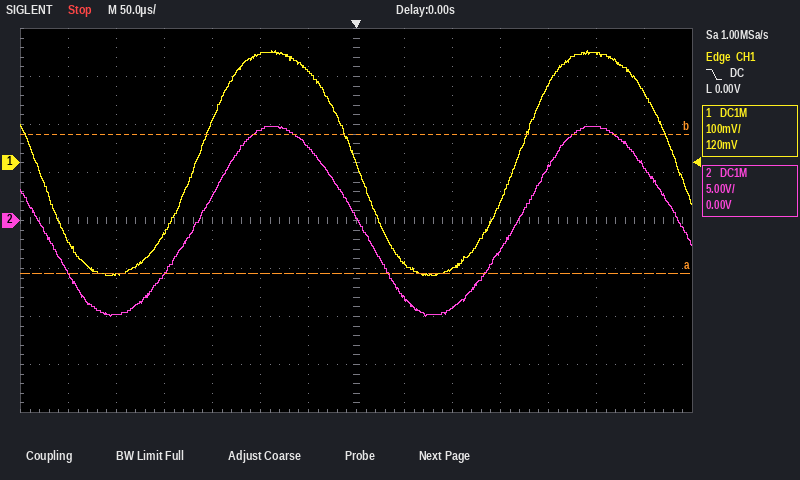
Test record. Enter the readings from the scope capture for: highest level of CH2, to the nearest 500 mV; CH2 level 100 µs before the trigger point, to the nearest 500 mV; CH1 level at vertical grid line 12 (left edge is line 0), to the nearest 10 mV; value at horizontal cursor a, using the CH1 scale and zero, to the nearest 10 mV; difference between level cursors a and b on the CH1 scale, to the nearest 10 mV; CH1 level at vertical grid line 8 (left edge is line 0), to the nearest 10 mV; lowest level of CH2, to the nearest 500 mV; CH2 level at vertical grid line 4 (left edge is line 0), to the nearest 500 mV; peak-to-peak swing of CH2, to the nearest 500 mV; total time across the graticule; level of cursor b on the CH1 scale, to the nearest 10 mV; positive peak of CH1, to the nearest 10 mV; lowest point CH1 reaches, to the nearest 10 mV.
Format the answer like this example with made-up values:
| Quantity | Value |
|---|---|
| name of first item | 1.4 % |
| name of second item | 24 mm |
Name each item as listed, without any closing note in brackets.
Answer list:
| Quantity | Value |
|---|---|
| highest level of CH2, to the nearest 500 mV | 10.0 V |
| CH2 level 100 µs before the trigger point, to the nearest 500 mV | 9.5 V |
| CH1 level at vertical grid line 12 (left edge is line 0), to the nearest 10 mV | 230 mV |
| value at horizontal cursor a, using the CH1 scale and zero, to the nearest 10 mV | -230 mV |
| difference between level cursors a and b on the CH1 scale, to the nearest 10 mV | 290 mV |
| CH1 level at vertical grid line 8 (left edge is line 0), to the nearest 10 mV | -210 mV |
| lowest level of CH2, to the nearest 500 mV | -10.0 V |
| CH2 level at vertical grid line 4 (left edge is line 0), to the nearest 500 mV | 2.5 V |
| peak-to-peak swing of CH2, to the nearest 500 mV | 20.0 V |
| total time across the graticule | 700 µs |
| level of cursor b on the CH1 scale, to the nearest 10 mV | 60 mV |
| positive peak of CH1, to the nearest 10 mV | 230 mV |
| lowest point CH1 reaches, to the nearest 10 mV | -230 mV |
